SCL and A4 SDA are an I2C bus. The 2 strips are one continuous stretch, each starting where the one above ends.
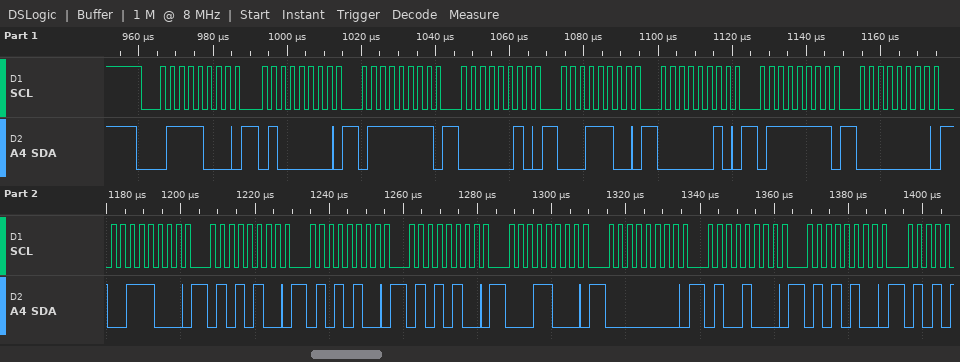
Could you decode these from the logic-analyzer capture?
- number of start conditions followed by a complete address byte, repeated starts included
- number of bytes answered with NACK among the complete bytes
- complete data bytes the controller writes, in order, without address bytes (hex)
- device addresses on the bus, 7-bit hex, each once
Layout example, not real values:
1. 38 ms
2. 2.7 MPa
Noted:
1. 1
2. 0
3. 40 7F 02 1C 02 7F 00 38 54 54 54 18 00 48 54
4. 0x3C
